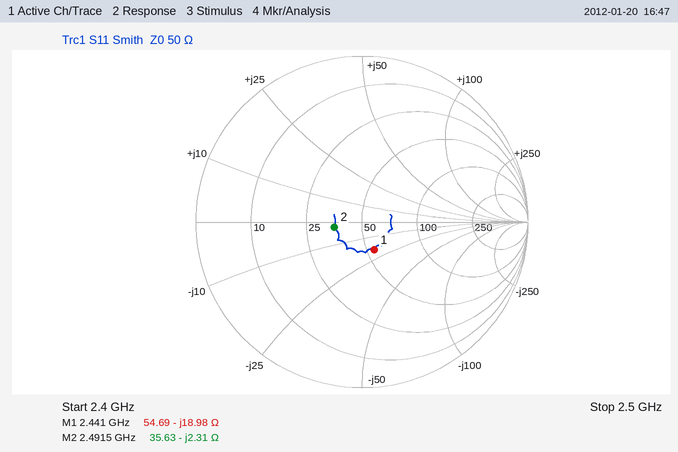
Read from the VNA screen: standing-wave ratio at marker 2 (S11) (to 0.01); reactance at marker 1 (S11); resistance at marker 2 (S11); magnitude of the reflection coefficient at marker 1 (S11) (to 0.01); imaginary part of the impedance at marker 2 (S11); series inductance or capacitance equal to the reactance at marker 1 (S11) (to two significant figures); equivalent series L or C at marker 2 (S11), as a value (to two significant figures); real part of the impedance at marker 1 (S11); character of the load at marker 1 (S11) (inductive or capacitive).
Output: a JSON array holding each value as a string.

["1.41", "-18.98 Ω", "35.63 Ω", "0.18", "-2.31 Ω", "3.4 pF", "28 pF", "54.69 Ω", "capacitive"]
